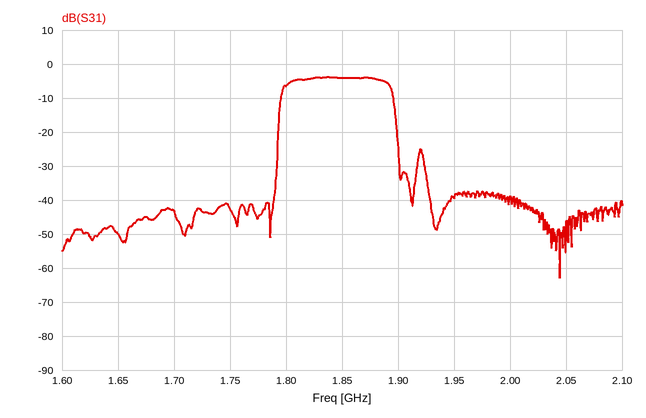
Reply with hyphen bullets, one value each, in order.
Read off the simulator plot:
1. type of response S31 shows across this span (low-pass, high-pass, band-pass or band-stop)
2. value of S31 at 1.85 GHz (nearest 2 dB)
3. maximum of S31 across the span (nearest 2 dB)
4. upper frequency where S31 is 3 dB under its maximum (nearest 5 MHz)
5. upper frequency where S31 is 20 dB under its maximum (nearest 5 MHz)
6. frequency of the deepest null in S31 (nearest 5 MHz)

- band-pass
- -4 dB
- -4 dB
- 1.895 GHz
- 1.900 GHz
- 2.045 GHz
